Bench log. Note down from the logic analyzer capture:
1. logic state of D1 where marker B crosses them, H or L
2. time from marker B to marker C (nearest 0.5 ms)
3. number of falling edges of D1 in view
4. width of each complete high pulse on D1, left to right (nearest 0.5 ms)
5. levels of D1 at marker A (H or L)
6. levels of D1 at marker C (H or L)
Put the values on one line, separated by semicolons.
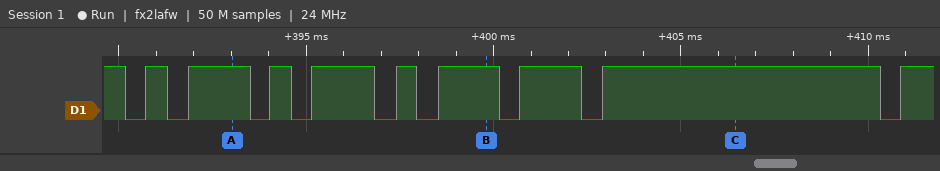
D1=H; 6.5 ms; 9; 0.5 ms, 1.5 ms, 0.5 ms, 1.5 ms, 0.5 ms, 1.5 ms, 1.5 ms, 7.5 ms; D1=H; D1=H
